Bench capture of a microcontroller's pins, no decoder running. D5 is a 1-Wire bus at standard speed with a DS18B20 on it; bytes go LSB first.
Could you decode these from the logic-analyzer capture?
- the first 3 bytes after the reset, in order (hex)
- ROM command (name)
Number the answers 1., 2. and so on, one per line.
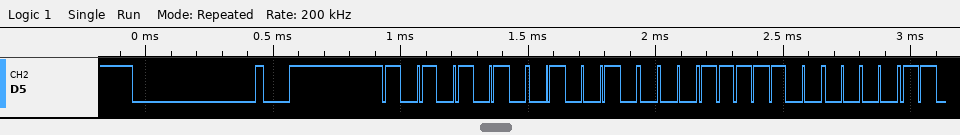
1. 55 12 3E
2. Match ROM
